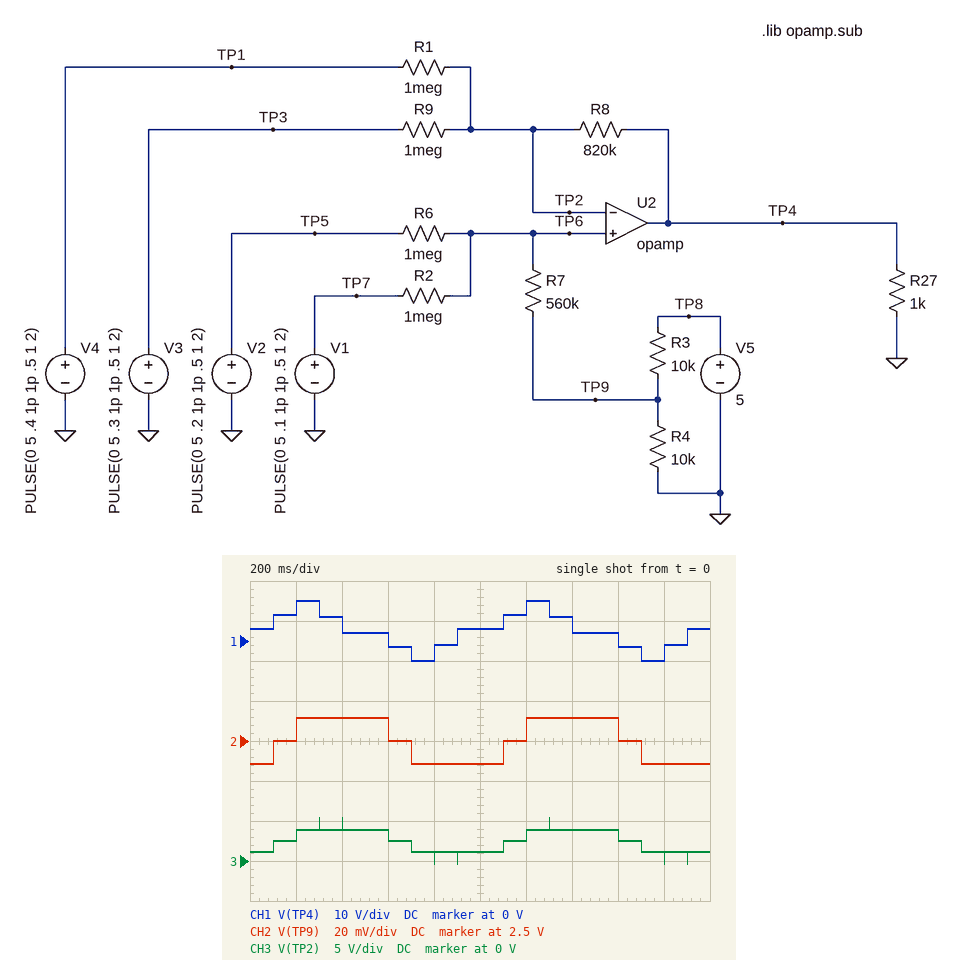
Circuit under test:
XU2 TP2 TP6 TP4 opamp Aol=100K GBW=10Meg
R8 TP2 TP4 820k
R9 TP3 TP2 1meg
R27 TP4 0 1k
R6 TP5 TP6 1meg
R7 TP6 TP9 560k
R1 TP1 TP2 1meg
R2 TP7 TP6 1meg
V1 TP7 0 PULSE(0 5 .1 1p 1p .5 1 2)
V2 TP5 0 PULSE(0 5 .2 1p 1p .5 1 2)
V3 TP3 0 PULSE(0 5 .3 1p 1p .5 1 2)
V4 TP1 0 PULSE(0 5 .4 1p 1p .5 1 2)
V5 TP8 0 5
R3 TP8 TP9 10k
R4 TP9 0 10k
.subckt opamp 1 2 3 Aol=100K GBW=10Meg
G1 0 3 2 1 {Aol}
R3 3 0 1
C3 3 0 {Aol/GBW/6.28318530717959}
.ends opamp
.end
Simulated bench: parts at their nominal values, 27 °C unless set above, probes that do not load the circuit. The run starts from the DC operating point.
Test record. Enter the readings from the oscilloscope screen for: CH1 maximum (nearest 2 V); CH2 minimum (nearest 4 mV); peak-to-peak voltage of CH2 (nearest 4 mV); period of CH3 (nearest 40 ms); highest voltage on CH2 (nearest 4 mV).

10 V
2.488 V
24 mV
1.00 s
2.512 V
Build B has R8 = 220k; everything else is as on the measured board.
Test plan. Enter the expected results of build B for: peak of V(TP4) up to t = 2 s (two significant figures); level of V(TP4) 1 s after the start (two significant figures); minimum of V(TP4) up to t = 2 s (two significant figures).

5.5 V
1.7 V
-510 mV
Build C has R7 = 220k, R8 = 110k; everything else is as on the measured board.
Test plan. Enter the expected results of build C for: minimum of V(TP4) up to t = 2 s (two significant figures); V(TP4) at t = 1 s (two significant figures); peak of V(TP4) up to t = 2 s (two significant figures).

1.0 V
2.1 V
4.0 V
